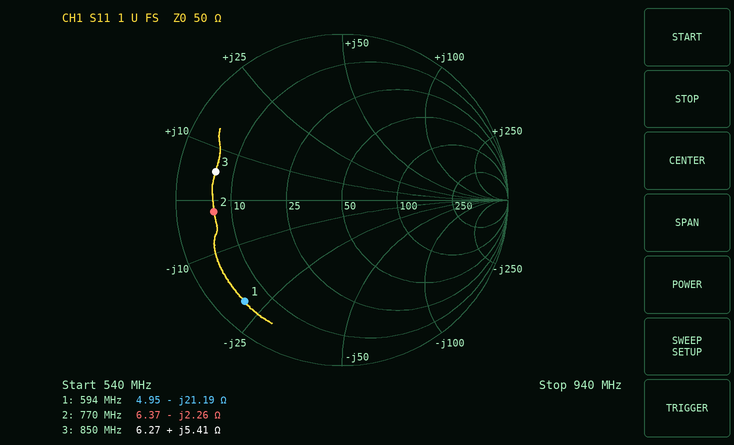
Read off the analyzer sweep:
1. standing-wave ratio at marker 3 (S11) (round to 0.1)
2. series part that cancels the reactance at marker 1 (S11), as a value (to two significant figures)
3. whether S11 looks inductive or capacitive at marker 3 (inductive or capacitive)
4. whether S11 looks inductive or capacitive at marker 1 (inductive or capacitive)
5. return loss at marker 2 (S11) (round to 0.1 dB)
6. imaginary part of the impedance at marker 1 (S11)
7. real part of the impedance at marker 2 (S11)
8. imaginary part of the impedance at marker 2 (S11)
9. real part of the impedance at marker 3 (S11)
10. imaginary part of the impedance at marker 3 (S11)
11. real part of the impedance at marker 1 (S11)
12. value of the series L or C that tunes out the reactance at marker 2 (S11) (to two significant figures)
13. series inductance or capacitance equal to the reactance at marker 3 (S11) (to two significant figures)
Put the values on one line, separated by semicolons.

8.1; 5.7 nH; inductive; capacitive; 2.2 dB; -21.19 Ω; 6.37 Ω; -2.26 Ω; 6.27 Ω; +5.41 Ω; 4.95 Ω; 470 pH; 1.0 nH
